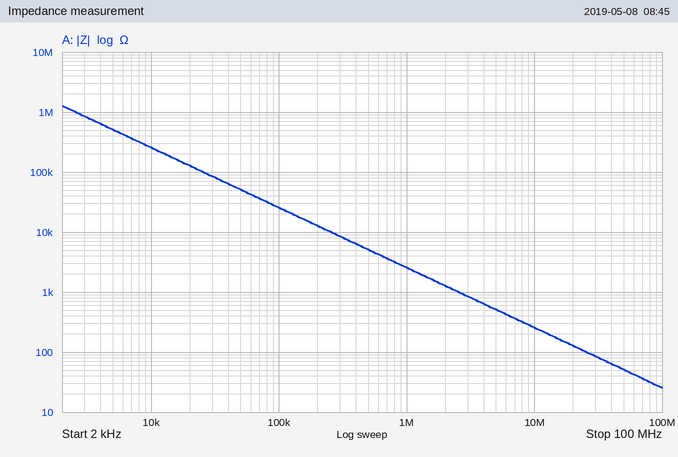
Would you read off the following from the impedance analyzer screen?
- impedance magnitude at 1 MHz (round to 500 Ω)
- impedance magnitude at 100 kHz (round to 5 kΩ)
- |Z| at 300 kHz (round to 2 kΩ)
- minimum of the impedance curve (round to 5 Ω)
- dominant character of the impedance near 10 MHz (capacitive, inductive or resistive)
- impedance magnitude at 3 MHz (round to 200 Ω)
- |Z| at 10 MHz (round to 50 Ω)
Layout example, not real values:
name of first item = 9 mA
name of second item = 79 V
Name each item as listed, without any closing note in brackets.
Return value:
impedance magnitude at 1 MHz = 2.5 kΩ
impedance magnitude at 100 kHz = 25 kΩ
|Z| at 300 kHz = 8 kΩ
minimum of the impedance curve = 25 Ω
dominant character of the impedance near 10 MHz = capacitive
impedance magnitude at 3 MHz = 800 Ω
|Z| at 10 MHz = 250 Ω
